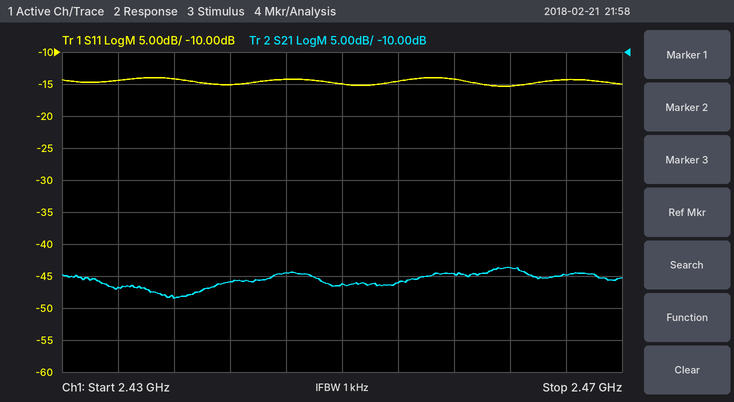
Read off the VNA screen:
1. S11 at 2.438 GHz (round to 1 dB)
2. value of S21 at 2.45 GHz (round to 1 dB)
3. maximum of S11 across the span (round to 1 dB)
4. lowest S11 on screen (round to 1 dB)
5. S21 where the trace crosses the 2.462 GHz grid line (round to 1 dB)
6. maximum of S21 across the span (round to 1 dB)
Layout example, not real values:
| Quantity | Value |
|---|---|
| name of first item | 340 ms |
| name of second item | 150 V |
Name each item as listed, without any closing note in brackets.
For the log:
| Quantity | Value |
|---|---|
| S11 at 2.438 GHz | -14 dB |
| value of S21 at 2.45 GHz | -46 dB |
| maximum of S11 across the span | -14 dB |
| lowest S11 on screen | -15 dB |
| S21 where the trace crosses the 2.462 GHz grid line | -44 dB |
| maximum of S21 across the span | -44 dB |
